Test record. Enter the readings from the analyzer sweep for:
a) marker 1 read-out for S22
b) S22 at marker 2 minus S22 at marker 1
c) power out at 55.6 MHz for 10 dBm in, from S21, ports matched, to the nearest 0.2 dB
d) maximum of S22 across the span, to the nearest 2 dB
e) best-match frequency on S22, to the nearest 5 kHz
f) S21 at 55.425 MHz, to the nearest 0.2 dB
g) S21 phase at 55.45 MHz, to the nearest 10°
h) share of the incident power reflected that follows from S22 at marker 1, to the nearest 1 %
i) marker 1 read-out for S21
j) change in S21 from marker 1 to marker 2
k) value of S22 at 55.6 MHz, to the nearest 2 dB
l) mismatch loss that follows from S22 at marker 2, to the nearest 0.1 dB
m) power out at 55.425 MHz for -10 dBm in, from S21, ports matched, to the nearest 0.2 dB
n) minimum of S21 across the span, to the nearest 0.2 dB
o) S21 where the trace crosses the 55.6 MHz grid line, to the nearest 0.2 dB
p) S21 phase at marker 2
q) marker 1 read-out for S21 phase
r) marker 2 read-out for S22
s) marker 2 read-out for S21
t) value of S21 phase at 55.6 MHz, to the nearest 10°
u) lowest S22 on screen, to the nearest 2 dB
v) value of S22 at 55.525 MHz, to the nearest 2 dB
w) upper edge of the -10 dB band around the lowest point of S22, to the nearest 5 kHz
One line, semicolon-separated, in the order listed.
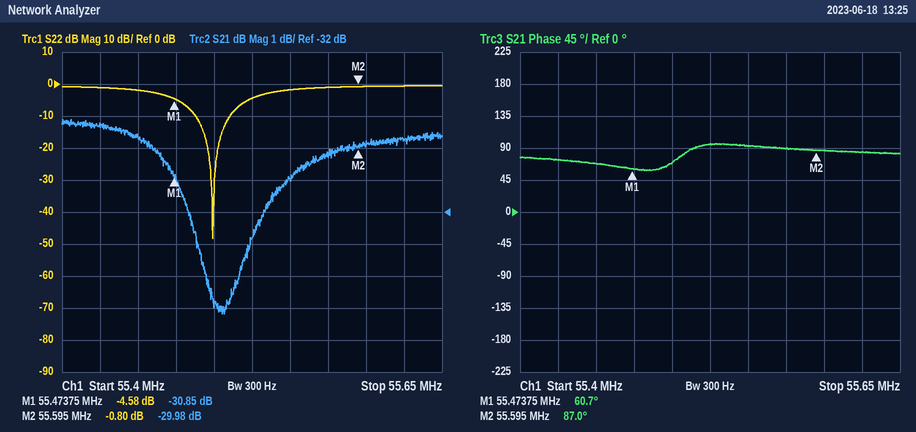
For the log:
-4.58 dB; 3.78 dB; -19.8 dBm; 0 dB; 55.500 MHz; -29.2 dB; 70°; 35 %; -30.85 dB; 0.87 dB; 0 dB; 7.7 dB; -39.2 dBm; -35.2 dB; -29.8 dB; 87.0°; 60.7°; -0.80 dB; -29.98 dB; 90°; -48 dB; -4 dB; 55.510 MHz
